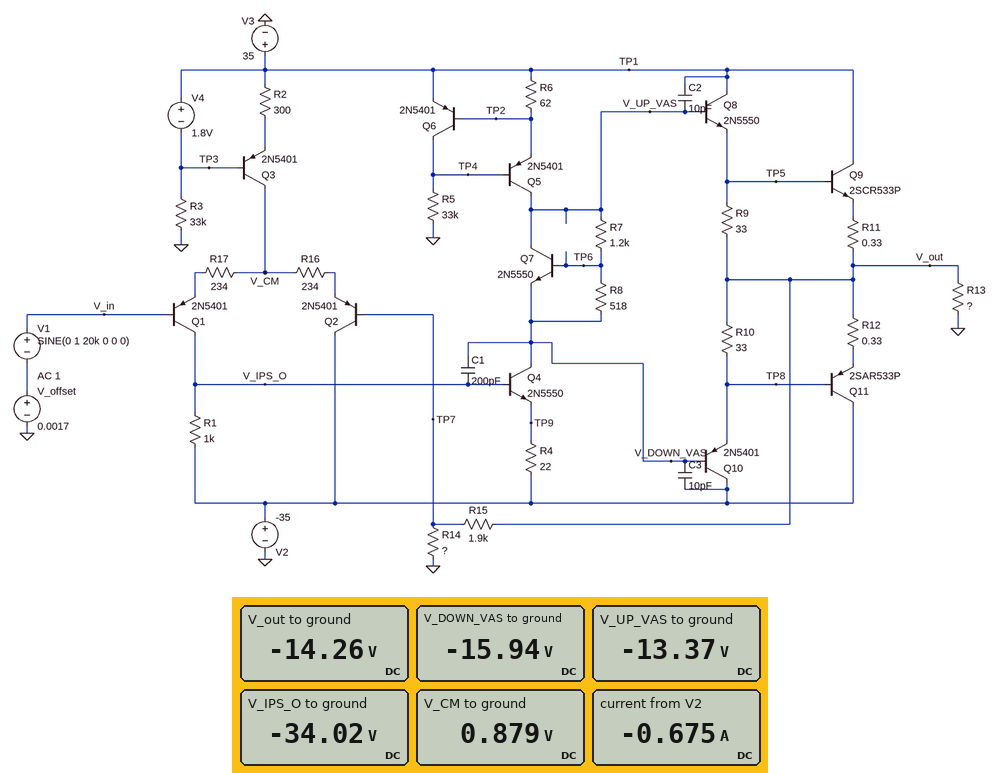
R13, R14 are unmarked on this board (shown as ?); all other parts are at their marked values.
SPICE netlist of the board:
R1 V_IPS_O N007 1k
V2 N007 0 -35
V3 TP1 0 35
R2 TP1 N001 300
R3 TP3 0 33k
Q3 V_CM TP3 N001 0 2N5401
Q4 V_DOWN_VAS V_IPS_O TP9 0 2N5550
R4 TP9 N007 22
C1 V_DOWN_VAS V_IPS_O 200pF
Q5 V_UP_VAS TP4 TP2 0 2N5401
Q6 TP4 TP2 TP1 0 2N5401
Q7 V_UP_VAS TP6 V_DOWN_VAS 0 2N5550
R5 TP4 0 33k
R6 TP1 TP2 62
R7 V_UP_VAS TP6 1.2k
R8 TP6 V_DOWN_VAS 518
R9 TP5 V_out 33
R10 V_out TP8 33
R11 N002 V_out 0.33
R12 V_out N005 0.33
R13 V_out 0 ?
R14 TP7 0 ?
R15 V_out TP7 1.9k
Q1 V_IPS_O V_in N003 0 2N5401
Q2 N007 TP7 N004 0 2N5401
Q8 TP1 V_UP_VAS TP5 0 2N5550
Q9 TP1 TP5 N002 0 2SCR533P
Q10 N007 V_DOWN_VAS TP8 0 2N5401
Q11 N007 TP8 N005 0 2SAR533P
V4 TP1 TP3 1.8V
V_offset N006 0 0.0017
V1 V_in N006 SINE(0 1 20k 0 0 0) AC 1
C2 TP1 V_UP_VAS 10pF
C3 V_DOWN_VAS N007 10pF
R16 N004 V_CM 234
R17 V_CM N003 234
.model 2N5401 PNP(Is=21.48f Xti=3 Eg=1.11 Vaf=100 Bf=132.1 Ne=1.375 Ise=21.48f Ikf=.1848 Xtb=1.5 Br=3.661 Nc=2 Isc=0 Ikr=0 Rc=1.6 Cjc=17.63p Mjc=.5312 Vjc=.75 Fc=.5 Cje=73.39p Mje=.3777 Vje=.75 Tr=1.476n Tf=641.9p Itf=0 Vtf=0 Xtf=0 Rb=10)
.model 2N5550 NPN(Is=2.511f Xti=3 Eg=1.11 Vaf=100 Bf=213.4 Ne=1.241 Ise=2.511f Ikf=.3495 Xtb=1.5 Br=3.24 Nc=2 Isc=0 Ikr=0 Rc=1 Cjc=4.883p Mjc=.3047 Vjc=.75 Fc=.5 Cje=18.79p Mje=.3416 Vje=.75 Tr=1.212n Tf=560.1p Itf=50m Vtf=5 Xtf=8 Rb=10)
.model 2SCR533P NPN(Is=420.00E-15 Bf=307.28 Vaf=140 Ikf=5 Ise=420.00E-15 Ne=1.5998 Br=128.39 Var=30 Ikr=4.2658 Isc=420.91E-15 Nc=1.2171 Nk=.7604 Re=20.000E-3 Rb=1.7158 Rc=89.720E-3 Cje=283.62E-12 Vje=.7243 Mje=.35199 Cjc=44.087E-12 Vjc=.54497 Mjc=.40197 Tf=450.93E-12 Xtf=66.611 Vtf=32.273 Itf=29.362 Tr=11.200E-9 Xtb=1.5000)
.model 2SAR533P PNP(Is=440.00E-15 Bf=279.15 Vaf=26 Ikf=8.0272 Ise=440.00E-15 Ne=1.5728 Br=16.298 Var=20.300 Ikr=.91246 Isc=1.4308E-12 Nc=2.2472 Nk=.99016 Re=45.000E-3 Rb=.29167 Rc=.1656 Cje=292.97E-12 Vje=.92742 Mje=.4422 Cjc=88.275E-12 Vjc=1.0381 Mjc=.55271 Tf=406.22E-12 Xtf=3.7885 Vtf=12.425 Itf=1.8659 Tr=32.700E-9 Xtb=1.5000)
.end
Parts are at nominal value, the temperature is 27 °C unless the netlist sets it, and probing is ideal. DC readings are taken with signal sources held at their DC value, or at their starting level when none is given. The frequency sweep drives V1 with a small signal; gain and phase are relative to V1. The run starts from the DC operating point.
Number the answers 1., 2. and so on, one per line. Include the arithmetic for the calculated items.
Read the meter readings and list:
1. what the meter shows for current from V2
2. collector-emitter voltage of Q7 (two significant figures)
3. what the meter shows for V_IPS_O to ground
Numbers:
1. -0.675 A
2. -13.37 V - (-15.94 V) = 2.6 V
3. -34.02 V
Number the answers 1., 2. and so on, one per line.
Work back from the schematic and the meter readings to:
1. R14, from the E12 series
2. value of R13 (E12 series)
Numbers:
1. 56 Ω
2. 22 Ω
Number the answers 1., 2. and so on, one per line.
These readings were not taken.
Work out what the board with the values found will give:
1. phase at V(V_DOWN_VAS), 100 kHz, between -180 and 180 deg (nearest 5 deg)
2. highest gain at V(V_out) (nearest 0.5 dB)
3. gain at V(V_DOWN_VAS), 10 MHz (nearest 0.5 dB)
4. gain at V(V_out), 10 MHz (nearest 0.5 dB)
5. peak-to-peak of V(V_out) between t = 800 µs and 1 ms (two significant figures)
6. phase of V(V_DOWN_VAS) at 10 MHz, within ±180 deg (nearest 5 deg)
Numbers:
1. -65 deg
2. 30.5 dB
3. -16.0 dB
4. -16.0 dB
5. 49 V
6. -130 deg
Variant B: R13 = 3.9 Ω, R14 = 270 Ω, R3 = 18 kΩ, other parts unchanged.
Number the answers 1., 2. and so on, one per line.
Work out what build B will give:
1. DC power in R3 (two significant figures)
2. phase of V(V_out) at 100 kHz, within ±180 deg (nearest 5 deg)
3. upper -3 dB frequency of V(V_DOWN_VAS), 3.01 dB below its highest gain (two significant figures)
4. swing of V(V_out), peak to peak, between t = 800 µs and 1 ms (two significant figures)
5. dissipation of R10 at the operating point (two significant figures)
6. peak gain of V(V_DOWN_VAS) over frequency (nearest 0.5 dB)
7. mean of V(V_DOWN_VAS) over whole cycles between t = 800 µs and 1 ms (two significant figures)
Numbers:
1. 61 mW
2. -30 deg
3. 170 kHz
4. 16 V
5. 32 mW
6. 19.0 dB
7. -5.0 V
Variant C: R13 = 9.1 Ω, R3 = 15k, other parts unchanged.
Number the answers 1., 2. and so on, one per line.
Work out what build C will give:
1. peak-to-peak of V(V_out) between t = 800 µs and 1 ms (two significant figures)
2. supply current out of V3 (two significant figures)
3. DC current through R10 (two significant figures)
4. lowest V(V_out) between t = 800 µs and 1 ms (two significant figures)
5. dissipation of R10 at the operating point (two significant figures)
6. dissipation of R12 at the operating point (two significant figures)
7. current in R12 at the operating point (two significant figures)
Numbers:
1. 48 V
2. 17 mA
3. 40 mA
4. -32 V
5. 52 mW
6. 770 mW
7. 1.5 A
